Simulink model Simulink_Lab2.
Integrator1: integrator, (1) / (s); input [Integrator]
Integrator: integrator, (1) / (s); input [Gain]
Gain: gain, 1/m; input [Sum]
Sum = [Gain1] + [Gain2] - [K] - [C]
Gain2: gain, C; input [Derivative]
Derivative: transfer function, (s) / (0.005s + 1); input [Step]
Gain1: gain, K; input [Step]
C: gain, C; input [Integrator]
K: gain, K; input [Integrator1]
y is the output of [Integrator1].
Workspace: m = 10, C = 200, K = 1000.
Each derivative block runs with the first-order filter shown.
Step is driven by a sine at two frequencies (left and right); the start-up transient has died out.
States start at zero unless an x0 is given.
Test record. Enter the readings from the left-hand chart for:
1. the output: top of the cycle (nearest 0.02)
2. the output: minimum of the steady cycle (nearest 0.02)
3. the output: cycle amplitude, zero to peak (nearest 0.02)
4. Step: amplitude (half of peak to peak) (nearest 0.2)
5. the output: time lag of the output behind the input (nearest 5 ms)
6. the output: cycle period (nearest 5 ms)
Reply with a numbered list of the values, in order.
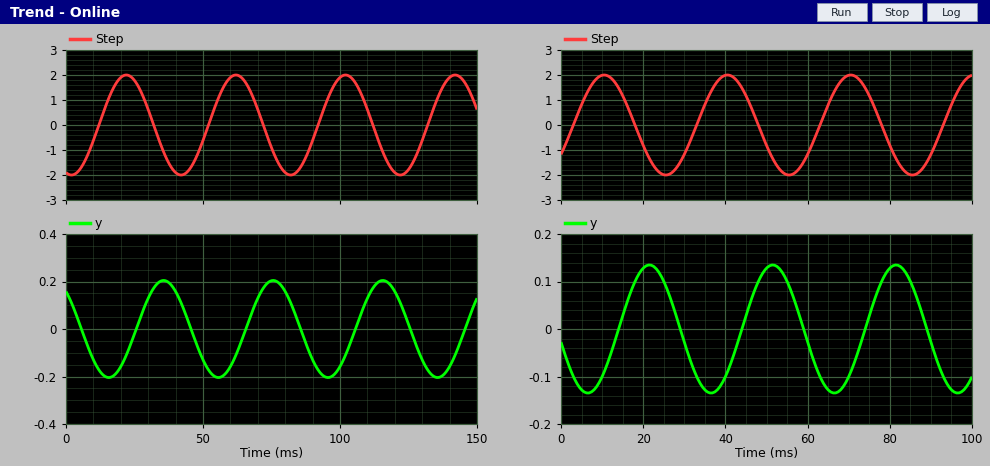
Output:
1. 0.20
2. -0.20
3. 0.20
4. 2.0
5. 15 ms
6. 40 ms
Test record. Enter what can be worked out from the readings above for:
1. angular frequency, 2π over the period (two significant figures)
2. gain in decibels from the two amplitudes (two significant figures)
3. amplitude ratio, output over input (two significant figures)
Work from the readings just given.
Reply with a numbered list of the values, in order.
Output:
1. 0.16 rad/ms
2. -20 dB
3. 0.10
